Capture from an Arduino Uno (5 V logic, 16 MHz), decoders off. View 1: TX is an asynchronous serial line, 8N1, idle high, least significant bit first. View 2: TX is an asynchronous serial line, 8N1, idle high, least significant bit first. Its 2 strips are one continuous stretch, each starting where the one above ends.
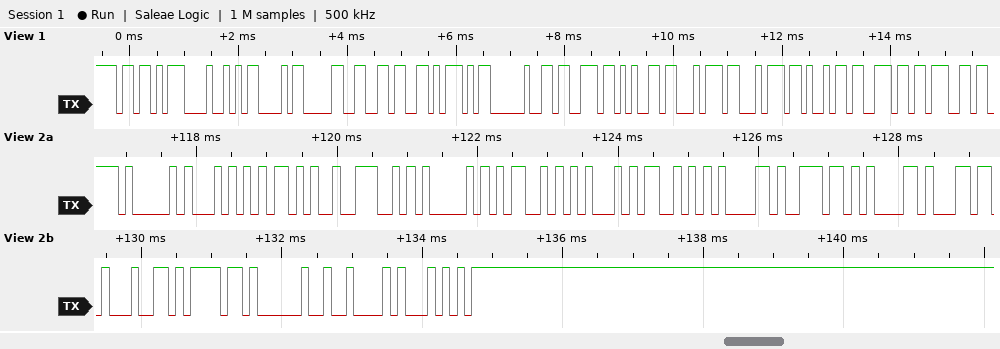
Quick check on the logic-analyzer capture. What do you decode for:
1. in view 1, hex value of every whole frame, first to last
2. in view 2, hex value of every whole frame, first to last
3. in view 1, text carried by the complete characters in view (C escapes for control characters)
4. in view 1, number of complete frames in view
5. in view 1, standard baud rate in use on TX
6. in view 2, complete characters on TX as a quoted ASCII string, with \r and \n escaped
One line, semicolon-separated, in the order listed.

5B 48 43 30 36 5D 20 73 65 74 74 69 6E 67; 41 54 2B 4E 41 4D 45 53 61 6E 61 6C 64 6F 20 42 54; "[HC06] setting"; 14; 9600 baud; "AT+NAMESanaldo BT"
